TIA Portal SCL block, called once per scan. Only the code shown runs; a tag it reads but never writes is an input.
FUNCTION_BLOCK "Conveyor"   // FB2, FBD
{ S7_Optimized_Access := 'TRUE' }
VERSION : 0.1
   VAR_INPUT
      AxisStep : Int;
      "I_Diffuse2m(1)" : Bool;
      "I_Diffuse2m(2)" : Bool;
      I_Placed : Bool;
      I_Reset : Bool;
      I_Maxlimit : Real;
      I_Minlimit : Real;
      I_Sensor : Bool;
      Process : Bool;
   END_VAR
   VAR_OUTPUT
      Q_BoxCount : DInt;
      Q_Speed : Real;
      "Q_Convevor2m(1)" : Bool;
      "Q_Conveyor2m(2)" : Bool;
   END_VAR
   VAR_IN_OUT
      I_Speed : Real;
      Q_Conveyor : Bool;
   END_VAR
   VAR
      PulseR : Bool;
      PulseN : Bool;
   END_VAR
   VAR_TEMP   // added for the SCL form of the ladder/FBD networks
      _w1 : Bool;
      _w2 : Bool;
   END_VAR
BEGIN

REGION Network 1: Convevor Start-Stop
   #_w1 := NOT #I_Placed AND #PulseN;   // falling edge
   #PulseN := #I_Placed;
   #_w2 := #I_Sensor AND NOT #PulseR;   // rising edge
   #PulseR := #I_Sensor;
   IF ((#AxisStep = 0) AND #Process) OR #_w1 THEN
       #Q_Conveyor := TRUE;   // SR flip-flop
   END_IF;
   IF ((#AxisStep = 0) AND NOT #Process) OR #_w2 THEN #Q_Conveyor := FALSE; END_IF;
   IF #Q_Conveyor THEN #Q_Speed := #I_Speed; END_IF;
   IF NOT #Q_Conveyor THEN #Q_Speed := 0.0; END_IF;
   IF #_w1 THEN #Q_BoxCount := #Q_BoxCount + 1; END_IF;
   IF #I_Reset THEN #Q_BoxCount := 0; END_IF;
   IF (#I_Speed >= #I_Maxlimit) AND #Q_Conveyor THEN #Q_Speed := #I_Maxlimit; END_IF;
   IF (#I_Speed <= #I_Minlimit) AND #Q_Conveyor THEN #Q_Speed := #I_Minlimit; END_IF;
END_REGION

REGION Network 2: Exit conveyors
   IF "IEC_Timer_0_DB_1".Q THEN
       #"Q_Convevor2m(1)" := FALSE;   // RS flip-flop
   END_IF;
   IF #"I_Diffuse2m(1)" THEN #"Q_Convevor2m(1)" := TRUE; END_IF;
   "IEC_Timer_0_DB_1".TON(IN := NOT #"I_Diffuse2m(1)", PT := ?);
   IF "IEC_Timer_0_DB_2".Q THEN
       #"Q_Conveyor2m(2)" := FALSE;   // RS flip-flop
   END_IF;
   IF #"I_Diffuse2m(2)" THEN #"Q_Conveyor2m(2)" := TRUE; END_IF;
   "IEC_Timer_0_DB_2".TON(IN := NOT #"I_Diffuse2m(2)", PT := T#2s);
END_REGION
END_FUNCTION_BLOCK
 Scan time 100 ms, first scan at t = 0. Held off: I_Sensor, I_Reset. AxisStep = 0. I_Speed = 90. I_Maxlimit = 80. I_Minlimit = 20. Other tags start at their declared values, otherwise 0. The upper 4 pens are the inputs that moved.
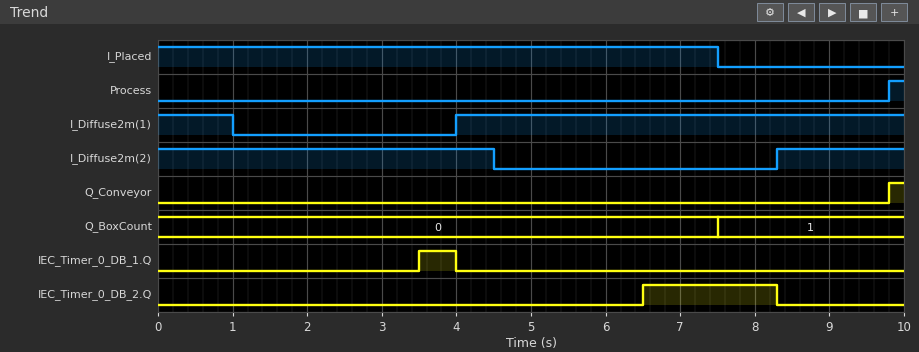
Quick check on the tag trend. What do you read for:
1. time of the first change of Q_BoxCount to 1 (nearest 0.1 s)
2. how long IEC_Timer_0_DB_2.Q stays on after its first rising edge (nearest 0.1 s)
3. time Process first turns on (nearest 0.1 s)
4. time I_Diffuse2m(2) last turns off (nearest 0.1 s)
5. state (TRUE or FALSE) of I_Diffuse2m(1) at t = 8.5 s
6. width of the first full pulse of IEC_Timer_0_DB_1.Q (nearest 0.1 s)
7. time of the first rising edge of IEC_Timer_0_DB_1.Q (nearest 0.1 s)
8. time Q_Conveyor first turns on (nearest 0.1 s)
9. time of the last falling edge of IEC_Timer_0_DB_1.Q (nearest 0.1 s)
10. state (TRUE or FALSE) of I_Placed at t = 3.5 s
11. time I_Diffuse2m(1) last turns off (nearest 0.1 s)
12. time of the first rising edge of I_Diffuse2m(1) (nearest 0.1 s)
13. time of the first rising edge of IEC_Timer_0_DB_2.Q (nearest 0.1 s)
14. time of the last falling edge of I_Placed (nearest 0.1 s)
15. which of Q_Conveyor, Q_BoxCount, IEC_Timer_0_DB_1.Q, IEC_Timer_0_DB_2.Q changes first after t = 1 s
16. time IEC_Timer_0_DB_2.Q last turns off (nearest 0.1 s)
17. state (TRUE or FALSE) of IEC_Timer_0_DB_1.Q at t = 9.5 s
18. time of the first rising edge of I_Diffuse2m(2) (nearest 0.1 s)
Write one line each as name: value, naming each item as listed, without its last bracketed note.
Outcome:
time of the first change of Q_BoxCount to 1: 7.5 s
how long IEC_Timer_0_DB_2.Q stays on after its first rising edge: 1.8 s
time Process first turns on: 9.8 s
time I_Diffuse2m(2) last turns off: 4.5 s
state (TRUE or FALSE) of I_Diffuse2m(1) at t = 8.5 s: TRUE
width of the first full pulse of IEC_Timer_0_DB_1.Q: 0.5 s
time of the first rising edge of IEC_Timer_0_DB_1.Q: 3.5 s
time Q_Conveyor first turns on: 9.8 s
time of the last falling edge of IEC_Timer_0_DB_1.Q: 4.0 s
state (TRUE or FALSE) of I_Placed at t = 3.5 s: TRUE
time I_Diffuse2m(1) last turns off: 1.0 s
time of the first rising edge of I_Diffuse2m(1): 4.0 s
time of the first rising edge of IEC_Timer_0_DB_2.Q: 6.5 s
time of the last falling edge of I_Placed: 7.5 s
which of Q_Conveyor, Q_BoxCount, IEC_Timer_0_DB_1.Q, IEC_Timer_0_DB_2.Q changes first after t = 1 s: IEC_Timer_0_DB_1.Q
time IEC_Timer_0_DB_2.Q last turns off: 8.3 s
state (TRUE or FALSE) of IEC_Timer_0_DB_1.Q at t = 9.5 s: FALSE
time of the first rising edge of I_Diffuse2m(2): 8.3 s
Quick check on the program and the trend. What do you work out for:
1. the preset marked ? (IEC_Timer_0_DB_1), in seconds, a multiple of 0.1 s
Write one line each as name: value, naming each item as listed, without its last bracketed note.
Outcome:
the preset marked ? (IEC_Timer_0_DB_1), in seconds, a multiple of 0.1 s: 2.5 s
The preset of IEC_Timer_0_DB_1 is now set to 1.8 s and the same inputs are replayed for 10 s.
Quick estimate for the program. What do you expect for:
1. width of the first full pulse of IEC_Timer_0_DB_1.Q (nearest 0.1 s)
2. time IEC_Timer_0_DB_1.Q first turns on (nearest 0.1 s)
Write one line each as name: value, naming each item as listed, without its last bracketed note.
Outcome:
width of the first full pulse of IEC_Timer_0_DB_1.Q: 1.2 s
time IEC_Timer_0_DB_1.Q first turns on: 2.8 s
